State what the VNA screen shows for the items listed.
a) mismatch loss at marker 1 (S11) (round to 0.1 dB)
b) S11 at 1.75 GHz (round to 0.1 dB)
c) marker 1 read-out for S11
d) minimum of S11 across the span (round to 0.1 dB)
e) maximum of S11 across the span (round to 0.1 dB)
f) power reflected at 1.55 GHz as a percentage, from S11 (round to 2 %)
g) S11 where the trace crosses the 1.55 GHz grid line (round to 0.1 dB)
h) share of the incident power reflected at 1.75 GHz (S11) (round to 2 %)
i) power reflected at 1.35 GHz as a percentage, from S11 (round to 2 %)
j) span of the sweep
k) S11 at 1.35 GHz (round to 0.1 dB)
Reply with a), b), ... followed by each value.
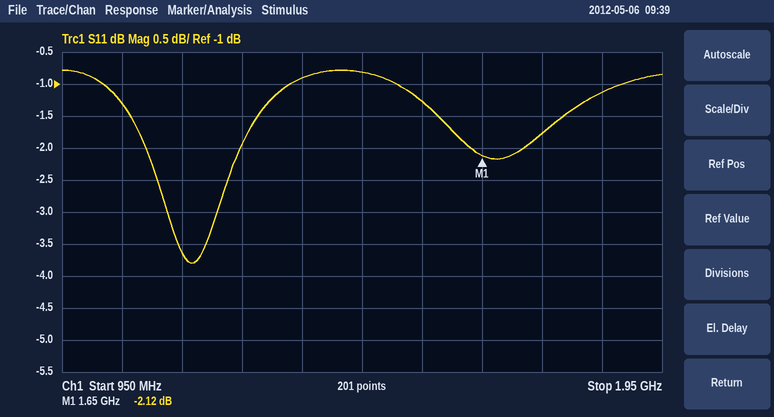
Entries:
a) 4.1 dB
b) -1.8 dB
c) -2.12 dB
d) -3.8 dB
e) -0.8 dB
f) 74 %
g) -1.3 dB
h) 66 %
i) 82 %
j) 1 GHz
k) -0.9 dB
